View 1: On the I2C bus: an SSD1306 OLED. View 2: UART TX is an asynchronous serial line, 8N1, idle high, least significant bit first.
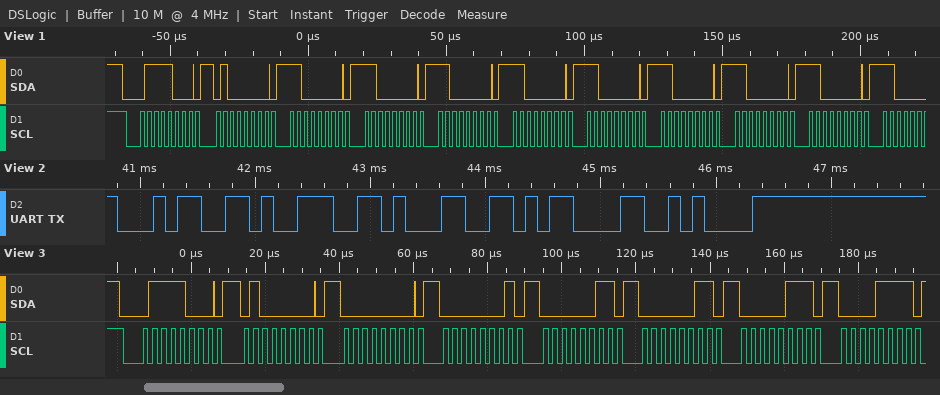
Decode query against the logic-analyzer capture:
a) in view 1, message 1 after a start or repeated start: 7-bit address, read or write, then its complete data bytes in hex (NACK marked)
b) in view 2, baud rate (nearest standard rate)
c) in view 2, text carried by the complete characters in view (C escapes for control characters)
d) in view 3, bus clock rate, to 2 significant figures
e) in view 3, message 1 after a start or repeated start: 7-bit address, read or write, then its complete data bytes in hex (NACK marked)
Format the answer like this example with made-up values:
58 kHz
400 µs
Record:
0x3C write: 40 C0 C0 C0 C0 C0 C0 C0 C0
9600 baud
"491\r\n"
400 kHz
0x3C write: 40 00 01 03 03 07 0F
